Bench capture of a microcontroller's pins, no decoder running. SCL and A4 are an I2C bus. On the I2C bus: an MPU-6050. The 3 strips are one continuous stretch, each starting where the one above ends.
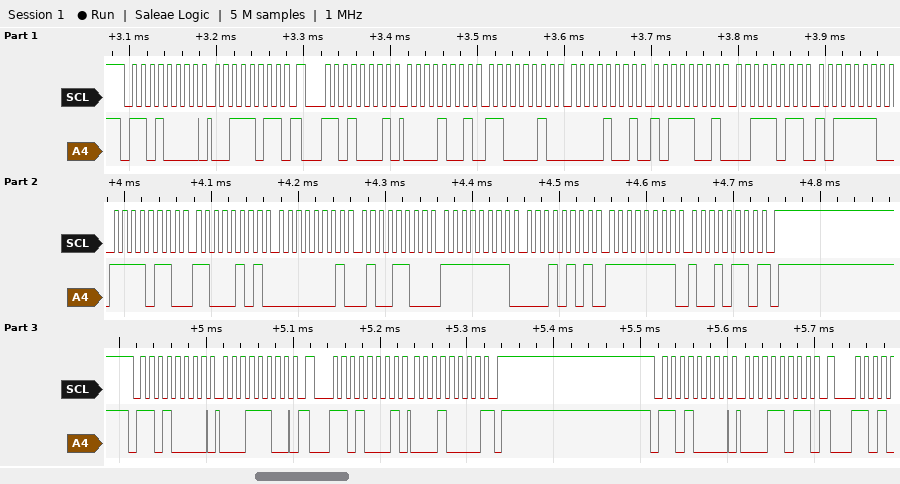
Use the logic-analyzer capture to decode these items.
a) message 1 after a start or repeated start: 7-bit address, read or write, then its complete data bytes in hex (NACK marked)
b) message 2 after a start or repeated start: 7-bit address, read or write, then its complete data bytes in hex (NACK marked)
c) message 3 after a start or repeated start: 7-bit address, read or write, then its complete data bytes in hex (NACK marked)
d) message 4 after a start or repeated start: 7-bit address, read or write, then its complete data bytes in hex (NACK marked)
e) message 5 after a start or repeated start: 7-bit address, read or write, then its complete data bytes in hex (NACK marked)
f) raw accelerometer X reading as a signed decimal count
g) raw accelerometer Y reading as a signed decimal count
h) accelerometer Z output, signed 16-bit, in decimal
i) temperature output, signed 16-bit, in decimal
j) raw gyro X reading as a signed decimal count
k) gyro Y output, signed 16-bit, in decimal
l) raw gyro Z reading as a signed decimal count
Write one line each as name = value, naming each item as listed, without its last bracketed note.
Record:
message 1 after a start or repeated start: 7-bit address, read or write, then its complete data bytes in hex = 0x68 write: 3B
message 2 after a start or repeated start: 7-bit address, read or write, then its complete data bytes in hex = 0x68 read: 09 C2 09 B9 3B BE F6 C5 01 4C FF 15 FF 96 NACK
message 3 after a start or repeated start: 7-bit address, read or write, then its complete data bytes in hex = 0x68 write: 1C
message 4 after a start or repeated start: 7-bit address, read or write, then its complete data bytes in hex = 0x68 read: 10 NACK
message 5 after a start or repeated start: 7-bit address, read or write, then its complete data bytes in hex = 0x68 write: 1B
raw accelerometer X reading as a signed decimal count = 2498
raw accelerometer Y reading as a signed decimal count = 2489
accelerometer Z output, signed 16-bit, in decimal = 15294
temperature output, signed 16-bit, in decimal = -2363
raw gyro X reading as a signed decimal count = 332
gyro Y output, signed 16-bit, in decimal = -235
raw gyro Z reading as a signed decimal count = -106
